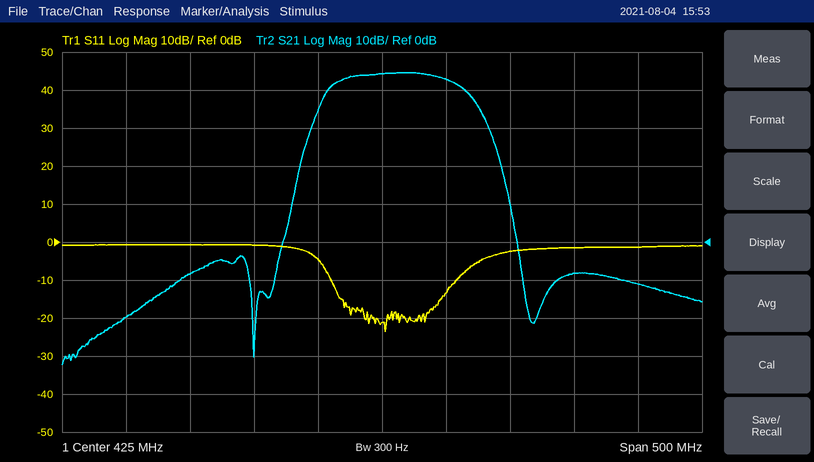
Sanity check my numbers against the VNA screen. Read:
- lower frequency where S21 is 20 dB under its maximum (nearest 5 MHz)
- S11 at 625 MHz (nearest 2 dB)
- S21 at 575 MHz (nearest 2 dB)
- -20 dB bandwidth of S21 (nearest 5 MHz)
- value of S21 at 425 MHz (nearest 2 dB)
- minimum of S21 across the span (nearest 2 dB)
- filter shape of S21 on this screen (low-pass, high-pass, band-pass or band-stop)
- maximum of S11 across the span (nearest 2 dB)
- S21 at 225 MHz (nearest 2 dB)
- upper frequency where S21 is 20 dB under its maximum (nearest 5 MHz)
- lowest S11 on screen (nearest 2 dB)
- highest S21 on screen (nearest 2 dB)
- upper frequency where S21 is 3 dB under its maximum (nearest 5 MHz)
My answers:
365 MHz
-2 dB
-8 dB
150 MHz
44 dB
-32 dB
band-pass
0 dB
-20 dB
515 MHz
-24 dB
44 dB
485 MHz
